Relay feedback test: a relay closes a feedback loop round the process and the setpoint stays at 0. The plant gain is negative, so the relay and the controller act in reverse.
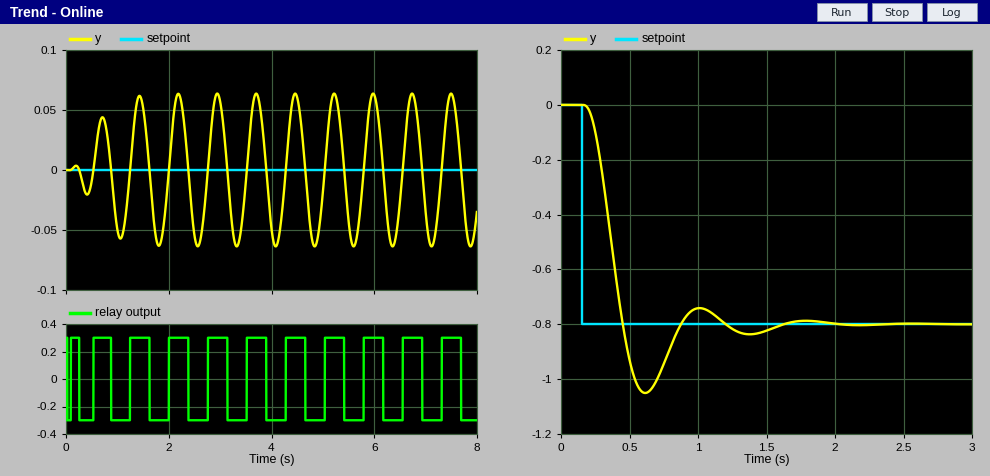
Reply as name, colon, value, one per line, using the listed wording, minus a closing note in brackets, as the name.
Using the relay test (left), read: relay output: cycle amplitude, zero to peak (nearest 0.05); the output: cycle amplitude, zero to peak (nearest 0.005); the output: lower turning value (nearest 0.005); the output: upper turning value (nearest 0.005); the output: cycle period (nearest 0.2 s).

relay output: cycle amplitude, zero to peak: 0.30
the output: cycle amplitude, zero to peak: 0.065
the output: lower turning value: -0.065
the output: upper turning value: 0.065
the output: cycle period: 0.8 s
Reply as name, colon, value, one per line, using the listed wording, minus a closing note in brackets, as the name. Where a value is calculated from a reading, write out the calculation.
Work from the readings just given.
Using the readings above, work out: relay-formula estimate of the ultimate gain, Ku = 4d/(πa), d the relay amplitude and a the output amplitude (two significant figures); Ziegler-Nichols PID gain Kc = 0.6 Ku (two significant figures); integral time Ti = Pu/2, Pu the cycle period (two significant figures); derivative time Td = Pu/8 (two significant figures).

relay-formula estimate of the ultimate gain, Ku = 4d/(πa), d the relay amplitude and a the output amplitude: 4 × 0.3 / (π × 0.065) = 5.9
Ziegler-Nichols PID gain Kc = 0.6 Ku: 0.6 × 5.9 = 3.5
integral time Ti = Pu/2, Pu the cycle period: 0.8 / 2 = 0.40 s
derivative time Td = Pu/8: 0.8 / 8 = 0.10 s
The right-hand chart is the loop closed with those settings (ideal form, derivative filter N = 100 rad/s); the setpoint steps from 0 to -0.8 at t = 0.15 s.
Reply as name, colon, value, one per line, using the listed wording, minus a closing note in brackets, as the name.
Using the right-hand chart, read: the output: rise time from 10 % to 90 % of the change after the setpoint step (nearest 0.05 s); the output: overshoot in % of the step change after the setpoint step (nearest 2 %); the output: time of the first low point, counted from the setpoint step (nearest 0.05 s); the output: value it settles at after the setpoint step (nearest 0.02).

the output: rise time from 10 % to 90 % of the change after the setpoint step: 0.20 s
the output: overshoot in % of the step change after the setpoint step: 32 %
the output: time of the first low point, counted from the setpoint step: 0.45 s
the output: value it settles at after the setpoint step: -0.80
